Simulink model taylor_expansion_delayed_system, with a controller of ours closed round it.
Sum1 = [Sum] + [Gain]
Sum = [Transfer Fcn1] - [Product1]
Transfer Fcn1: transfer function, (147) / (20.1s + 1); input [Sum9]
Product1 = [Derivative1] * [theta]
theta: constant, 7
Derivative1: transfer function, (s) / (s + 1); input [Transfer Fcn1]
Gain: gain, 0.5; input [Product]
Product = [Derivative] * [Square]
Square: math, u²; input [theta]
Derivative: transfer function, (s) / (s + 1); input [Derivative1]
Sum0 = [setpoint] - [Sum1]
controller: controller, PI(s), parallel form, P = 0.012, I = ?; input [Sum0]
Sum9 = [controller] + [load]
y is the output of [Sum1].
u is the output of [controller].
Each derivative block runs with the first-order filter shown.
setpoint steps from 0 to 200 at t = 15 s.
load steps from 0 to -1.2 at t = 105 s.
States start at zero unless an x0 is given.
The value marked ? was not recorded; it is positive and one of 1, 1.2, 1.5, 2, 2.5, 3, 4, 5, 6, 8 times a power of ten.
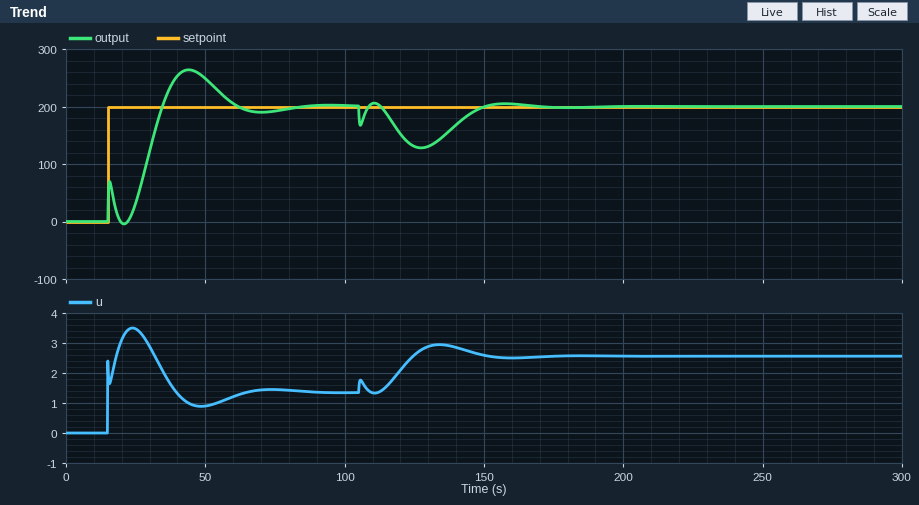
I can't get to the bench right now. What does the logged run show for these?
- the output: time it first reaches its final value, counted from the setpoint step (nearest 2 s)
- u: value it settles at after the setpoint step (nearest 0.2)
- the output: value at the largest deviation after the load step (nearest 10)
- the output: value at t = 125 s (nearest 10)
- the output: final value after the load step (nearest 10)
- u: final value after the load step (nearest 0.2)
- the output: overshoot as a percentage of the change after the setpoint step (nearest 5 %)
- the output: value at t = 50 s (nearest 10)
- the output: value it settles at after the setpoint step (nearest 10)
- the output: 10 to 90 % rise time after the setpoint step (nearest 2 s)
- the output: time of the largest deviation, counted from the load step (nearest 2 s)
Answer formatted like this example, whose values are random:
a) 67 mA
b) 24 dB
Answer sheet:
a) 20 s
b) 1.4
c) 130
d) 130
e) 200
f) 2.6
g) 30 %
h) 250
i) 200
j) 18 s
k) 22 s
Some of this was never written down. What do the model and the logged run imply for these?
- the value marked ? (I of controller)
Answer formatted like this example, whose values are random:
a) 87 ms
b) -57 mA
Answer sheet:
a) 0.0008
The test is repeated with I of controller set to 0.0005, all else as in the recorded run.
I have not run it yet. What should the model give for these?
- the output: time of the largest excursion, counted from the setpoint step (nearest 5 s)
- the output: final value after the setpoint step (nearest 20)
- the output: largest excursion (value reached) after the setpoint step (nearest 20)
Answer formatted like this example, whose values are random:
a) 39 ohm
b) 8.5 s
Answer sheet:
a) 30 s
b) 200
c) 220
